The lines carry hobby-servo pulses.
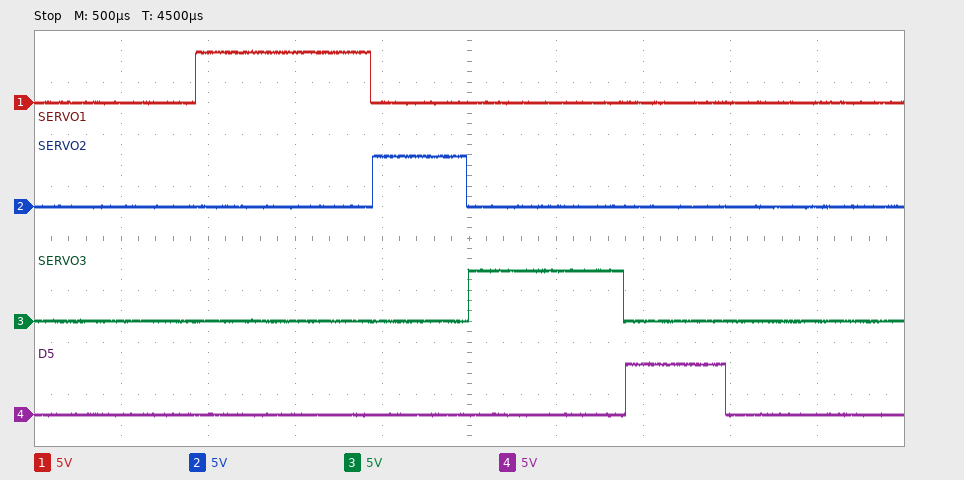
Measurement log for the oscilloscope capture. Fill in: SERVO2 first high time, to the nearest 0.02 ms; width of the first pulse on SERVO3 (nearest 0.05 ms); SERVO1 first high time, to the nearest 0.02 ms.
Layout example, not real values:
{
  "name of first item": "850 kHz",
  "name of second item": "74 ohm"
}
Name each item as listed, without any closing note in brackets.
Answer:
{
  "SERVO2 first high time, to the nearest 0.02 ms": "0.54 ms",
  "width of the first pulse on SERVO3": "0.90 ms",
  "SERVO1 first high time, to the nearest 0.02 ms": "1.00 ms"
}
